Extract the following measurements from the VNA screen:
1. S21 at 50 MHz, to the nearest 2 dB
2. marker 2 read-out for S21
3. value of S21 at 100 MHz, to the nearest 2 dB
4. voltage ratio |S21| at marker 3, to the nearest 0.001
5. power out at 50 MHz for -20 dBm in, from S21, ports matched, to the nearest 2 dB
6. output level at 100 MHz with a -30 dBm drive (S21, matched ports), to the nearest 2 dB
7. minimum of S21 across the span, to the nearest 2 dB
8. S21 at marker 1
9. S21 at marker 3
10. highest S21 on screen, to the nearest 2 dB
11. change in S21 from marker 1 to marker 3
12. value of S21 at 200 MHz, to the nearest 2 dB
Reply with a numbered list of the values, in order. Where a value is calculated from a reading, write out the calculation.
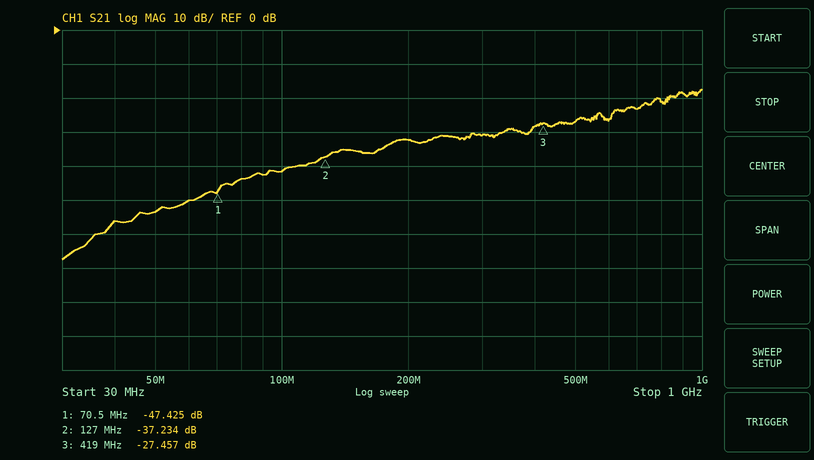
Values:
1. -54 dB
2. -37.234 dB
3. -42 dB
4. 10^(-27.457/20) ≈ 0.042
5. -20 dBm + (-54 dB) = -74 dBm
6. -30 dBm + (-42 dB) = -72 dBm
7. -68 dB
8. -47.425 dB
9. -27.457 dB
10. -18 dB
11. -27.457 − (-47.425) = 19.968 dB
12. -32 dB
